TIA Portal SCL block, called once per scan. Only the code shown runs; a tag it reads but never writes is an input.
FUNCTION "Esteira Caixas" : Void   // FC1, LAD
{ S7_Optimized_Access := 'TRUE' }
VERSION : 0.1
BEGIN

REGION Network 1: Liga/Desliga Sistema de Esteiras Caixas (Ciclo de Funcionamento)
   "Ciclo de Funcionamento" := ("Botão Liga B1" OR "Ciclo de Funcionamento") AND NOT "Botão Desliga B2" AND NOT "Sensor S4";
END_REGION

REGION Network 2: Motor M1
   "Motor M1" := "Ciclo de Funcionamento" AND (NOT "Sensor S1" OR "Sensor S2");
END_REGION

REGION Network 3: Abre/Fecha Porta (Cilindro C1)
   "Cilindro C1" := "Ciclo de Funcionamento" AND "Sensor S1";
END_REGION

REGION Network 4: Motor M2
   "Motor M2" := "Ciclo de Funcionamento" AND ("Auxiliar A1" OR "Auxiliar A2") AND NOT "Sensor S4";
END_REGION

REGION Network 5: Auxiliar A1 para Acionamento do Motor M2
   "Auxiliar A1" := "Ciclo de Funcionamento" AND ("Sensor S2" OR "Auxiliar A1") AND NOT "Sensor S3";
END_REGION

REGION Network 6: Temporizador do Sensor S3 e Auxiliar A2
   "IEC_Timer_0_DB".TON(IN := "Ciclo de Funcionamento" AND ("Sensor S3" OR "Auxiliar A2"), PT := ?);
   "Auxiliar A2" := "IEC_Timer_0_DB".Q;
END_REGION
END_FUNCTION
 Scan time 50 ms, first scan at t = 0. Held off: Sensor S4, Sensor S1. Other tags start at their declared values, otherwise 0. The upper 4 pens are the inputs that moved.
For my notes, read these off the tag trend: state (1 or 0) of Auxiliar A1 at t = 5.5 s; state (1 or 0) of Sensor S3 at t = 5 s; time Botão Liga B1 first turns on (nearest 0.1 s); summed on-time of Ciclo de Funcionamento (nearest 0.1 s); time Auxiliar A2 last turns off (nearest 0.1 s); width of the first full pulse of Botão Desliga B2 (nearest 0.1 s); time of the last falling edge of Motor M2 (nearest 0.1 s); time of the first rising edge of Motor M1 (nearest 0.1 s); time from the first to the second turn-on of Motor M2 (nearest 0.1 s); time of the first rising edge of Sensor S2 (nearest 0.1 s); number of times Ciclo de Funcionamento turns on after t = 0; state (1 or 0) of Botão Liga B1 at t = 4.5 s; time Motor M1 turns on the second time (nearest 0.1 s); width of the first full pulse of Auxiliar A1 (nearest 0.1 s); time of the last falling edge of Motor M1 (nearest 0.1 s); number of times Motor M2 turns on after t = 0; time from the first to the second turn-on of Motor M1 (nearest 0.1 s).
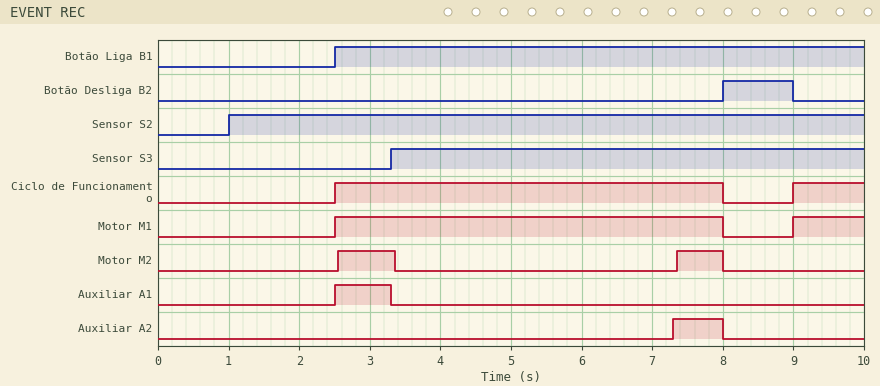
0
1
2.5 s
6.5 s
8.0 s
1.0 s
8.0 s
2.5 s
4.8 s
1.0 s
2
1
9.0 s
0.8 s
8.0 s
2
6.5 s
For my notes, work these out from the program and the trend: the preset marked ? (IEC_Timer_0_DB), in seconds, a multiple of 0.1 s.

4.0 s
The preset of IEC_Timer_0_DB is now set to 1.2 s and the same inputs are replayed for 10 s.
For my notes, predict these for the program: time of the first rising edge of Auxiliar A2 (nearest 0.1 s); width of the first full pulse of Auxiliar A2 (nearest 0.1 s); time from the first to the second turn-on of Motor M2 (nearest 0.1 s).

4.5 s
3.5 s
2.0 s
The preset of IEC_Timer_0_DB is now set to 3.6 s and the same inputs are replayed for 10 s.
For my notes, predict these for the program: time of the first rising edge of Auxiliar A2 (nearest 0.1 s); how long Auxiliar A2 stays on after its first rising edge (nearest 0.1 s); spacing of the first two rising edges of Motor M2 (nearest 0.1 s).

6.9 s
1.1 s
4.4 s
